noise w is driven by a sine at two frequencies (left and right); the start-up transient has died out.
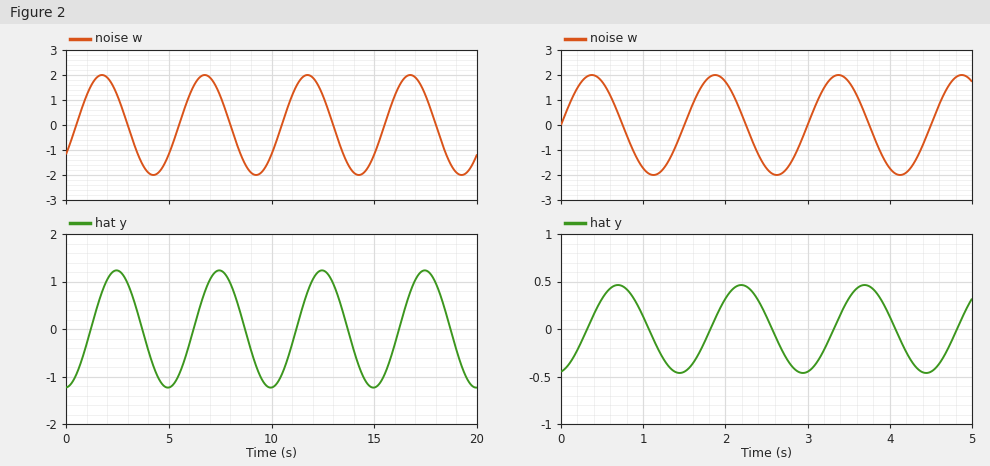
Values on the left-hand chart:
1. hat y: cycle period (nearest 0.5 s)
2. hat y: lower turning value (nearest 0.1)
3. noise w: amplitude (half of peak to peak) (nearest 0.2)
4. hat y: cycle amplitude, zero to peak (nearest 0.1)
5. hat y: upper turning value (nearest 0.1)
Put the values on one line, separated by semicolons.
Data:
5.0 s; -1.2; 2.0; 1.2; 1.2
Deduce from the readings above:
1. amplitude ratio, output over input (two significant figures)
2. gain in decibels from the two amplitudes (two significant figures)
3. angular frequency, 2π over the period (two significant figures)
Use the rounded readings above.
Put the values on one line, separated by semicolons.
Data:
0.60; -4.4 dB; 1.3 rad/s
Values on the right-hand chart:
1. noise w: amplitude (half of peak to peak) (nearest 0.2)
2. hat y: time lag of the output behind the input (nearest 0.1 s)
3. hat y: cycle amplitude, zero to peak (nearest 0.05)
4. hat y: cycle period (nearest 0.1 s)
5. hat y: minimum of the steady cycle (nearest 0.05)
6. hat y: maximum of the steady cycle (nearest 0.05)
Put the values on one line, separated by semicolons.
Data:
2.0; 0.3 s; 0.45; 1.5 s; -0.45; 0.45
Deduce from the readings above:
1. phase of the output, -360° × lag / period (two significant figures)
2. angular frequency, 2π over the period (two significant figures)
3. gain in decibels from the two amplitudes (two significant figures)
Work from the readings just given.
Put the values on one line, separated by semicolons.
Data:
-72°; 4.2 rad/s; -13 dB
